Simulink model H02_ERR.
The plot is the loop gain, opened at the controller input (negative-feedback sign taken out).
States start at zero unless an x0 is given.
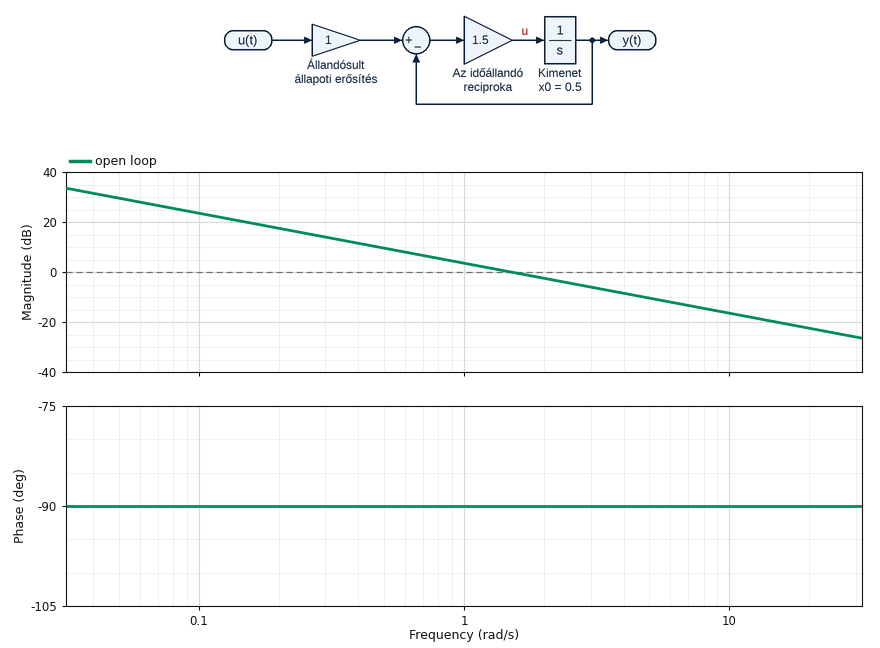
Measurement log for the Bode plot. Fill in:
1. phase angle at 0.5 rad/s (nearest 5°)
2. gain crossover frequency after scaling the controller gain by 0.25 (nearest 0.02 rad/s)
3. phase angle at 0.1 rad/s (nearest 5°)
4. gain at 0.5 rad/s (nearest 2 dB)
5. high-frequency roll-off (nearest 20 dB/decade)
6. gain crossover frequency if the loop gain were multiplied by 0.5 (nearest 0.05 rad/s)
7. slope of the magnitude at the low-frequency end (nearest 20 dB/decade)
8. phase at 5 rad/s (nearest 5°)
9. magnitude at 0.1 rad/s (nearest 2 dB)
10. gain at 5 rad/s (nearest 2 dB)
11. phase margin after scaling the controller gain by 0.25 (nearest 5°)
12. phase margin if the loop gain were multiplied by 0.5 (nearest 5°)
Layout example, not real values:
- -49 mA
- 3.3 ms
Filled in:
- -90°
- 0.38 rad/s
- -90°
- 10 dB
- -20 dB/decade
- 0.75 rad/s
- -20 dB/decade
- -90°
- 24 dB
- -10 dB
- 90°
- 90°
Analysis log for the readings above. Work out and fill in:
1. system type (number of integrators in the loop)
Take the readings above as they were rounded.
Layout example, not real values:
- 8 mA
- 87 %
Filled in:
- 1
